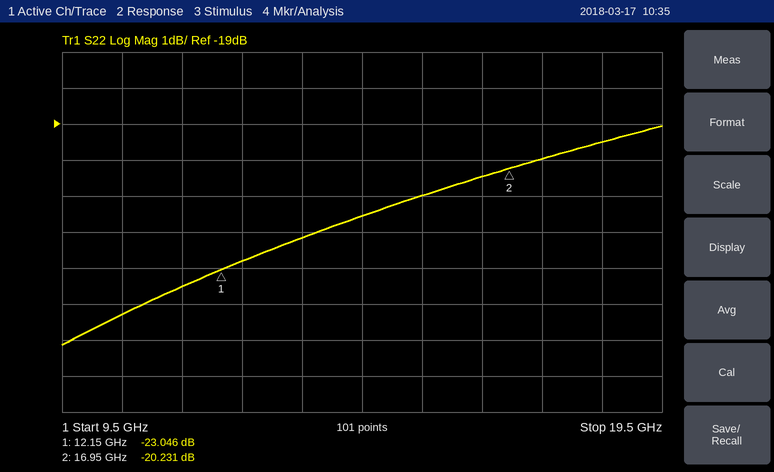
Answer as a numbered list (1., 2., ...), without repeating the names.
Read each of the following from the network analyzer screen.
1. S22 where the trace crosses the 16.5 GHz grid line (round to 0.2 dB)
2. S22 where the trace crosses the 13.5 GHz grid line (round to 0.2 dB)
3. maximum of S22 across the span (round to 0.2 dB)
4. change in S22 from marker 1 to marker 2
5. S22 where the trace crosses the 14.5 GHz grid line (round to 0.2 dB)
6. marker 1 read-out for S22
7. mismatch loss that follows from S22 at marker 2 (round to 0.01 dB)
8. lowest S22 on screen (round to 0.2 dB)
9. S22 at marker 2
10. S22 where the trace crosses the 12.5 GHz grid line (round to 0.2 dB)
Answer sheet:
1. -20.4 dB
2. -22.2 dB
3. -19.0 dB
4. 2.815 dB
5. -21.6 dB
6. -23.046 dB
7. 0.04 dB
8. -25.2 dB
9. -20.231 dB
10. -22.8 dB
